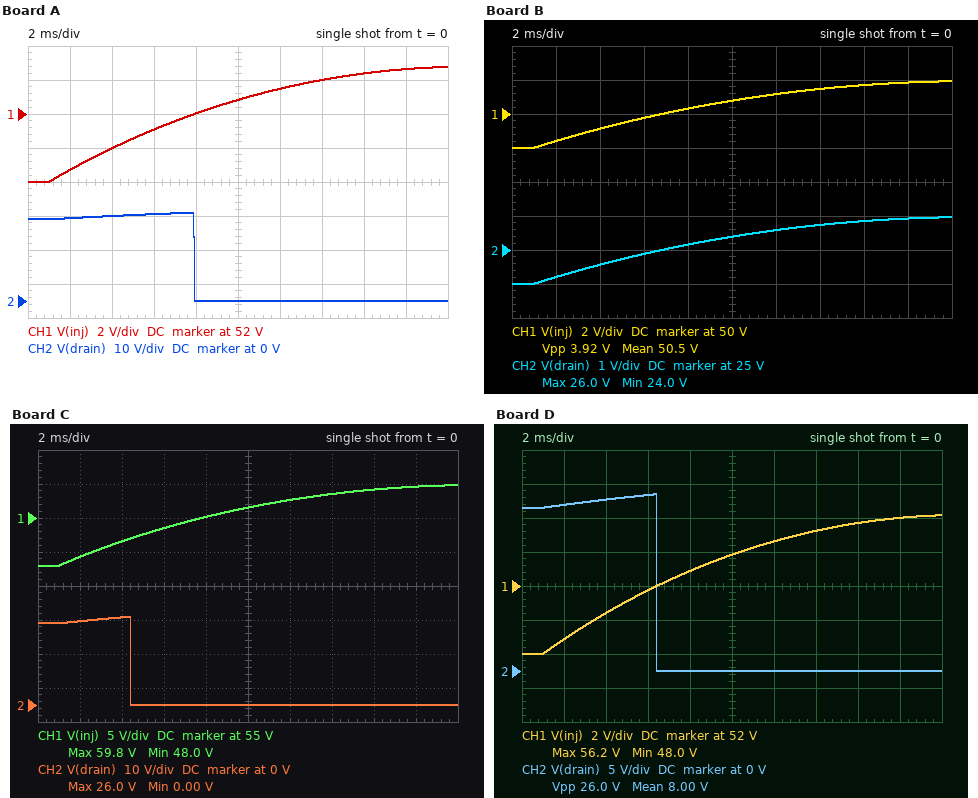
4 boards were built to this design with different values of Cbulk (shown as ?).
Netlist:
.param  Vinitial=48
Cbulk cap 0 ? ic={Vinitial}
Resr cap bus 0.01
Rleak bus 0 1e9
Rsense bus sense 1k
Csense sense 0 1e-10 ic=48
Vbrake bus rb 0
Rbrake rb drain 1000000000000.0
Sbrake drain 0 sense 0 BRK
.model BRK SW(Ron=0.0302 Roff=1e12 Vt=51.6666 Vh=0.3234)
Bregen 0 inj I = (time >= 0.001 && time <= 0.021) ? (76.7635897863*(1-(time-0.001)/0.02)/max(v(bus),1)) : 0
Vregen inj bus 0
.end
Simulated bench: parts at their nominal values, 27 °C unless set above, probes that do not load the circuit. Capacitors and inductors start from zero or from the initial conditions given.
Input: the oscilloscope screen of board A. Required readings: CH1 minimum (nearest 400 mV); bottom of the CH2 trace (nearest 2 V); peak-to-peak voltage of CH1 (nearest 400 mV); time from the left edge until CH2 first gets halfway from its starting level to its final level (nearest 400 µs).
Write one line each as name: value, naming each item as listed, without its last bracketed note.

CH1 minimum: 48.0 V
bottom of the CH2 trace: 0 V
peak-to-peak voltage of CH1: 6.8 V
time from the left edge until CH2 first gets halfway from its starting level to its final level: 8.0 ms
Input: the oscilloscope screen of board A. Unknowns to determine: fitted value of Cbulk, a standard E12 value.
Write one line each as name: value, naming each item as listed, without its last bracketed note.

fitted value of Cbulk, a standard E12 value: 2.2 mF
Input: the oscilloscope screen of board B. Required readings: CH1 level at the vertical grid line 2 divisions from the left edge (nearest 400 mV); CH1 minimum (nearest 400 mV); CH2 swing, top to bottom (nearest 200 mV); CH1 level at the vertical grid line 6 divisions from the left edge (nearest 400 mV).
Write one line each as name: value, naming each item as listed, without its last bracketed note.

CH1 level at the vertical grid line 2 divisions from the left edge: 49.2 V
CH1 minimum: 48.0 V
CH2 swing, top to bottom: 2.0 V
CH1 level at the vertical grid line 6 divisions from the left edge: 51.2 V
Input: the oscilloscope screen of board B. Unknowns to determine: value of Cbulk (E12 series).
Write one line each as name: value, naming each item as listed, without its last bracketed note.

value of Cbulk: 3.9 mF
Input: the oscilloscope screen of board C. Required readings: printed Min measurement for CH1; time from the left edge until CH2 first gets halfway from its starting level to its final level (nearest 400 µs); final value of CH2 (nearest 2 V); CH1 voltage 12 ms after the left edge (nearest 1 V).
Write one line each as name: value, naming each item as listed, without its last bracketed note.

printed Min measurement for CH1: 48.0 V
time from the left edge until CH2 first gets halfway from its starting level to its final level: 4.4 ms
final value of CH2: 0 V
CH1 voltage 12 ms after the left edge: 58 V
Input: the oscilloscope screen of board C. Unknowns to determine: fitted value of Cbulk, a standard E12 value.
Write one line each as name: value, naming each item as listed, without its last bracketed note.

fitted value of Cbulk, a standard E12 value: 1.2 mF
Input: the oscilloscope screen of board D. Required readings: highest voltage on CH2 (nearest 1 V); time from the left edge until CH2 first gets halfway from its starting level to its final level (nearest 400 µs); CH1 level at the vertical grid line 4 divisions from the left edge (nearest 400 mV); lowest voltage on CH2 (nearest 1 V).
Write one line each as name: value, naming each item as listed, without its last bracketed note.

highest voltage on CH2: 26 V
time from the left edge until CH2 first gets halfway from its starting level to its final level: 6.4 ms
CH1 level at the vertical grid line 4 divisions from the left edge: 52.8 V
lowest voltage on CH2: 0 V
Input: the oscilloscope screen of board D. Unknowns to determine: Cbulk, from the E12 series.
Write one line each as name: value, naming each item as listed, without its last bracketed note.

Cbulk, from the E12 series: 1.8 mF
